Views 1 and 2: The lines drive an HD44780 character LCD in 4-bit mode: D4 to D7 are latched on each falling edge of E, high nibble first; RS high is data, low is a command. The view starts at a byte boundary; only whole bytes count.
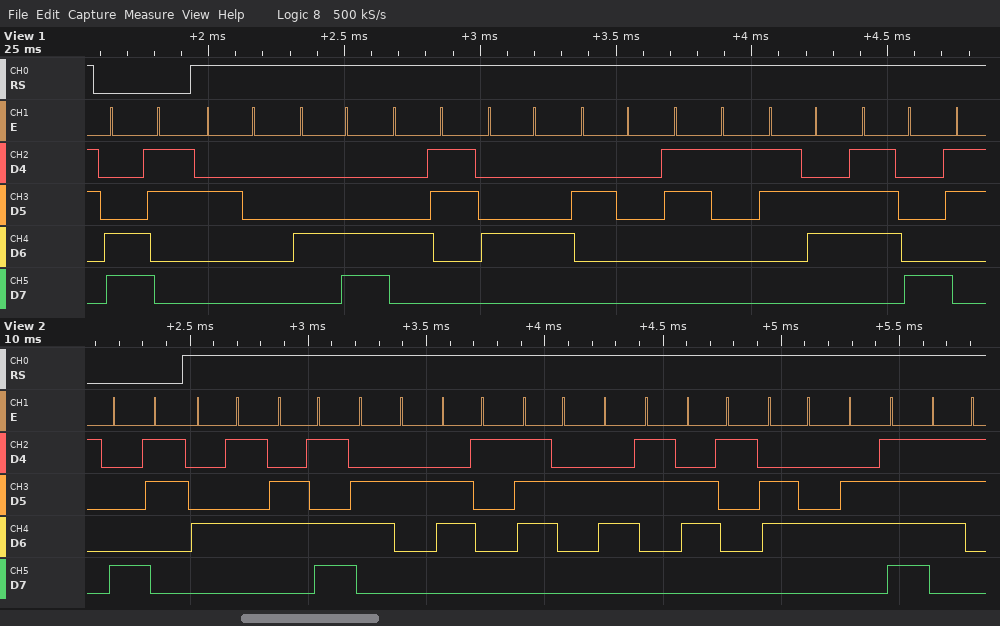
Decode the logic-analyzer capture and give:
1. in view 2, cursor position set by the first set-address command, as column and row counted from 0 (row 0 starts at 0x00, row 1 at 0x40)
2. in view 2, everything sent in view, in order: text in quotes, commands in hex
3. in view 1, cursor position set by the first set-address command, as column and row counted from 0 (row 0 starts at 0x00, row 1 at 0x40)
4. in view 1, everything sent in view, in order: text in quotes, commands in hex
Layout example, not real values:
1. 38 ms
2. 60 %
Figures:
1. column 3, row 0
2. 0x83 "Embarcados"
3. column 3, row 1
4. 0xC3 " LCD 16x"
